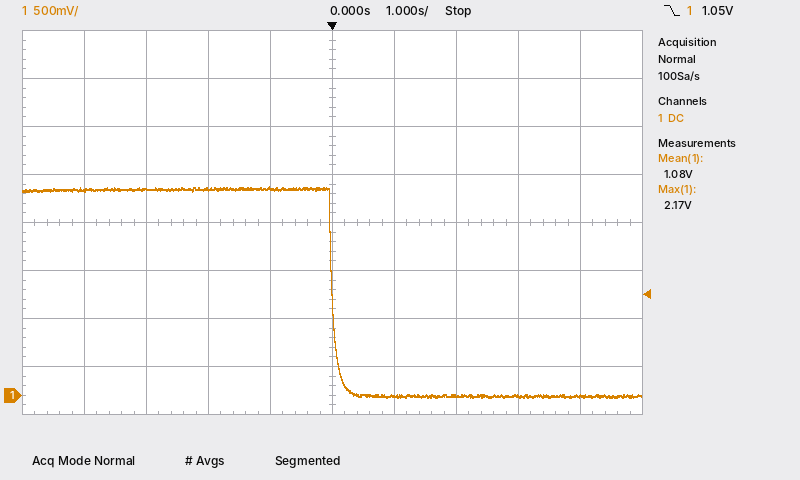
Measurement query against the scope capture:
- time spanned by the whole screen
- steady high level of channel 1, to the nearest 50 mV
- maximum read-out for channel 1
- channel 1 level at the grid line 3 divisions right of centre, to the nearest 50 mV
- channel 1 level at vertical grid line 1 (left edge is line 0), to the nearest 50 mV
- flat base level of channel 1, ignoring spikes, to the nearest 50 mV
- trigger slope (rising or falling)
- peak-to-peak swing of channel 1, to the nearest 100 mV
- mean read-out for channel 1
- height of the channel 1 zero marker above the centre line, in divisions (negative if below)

10 s
2.15 V
2.17 V
0 mV
2.15 V
0 mV
falling
2.20 V
1.08 V
-3.6 div
